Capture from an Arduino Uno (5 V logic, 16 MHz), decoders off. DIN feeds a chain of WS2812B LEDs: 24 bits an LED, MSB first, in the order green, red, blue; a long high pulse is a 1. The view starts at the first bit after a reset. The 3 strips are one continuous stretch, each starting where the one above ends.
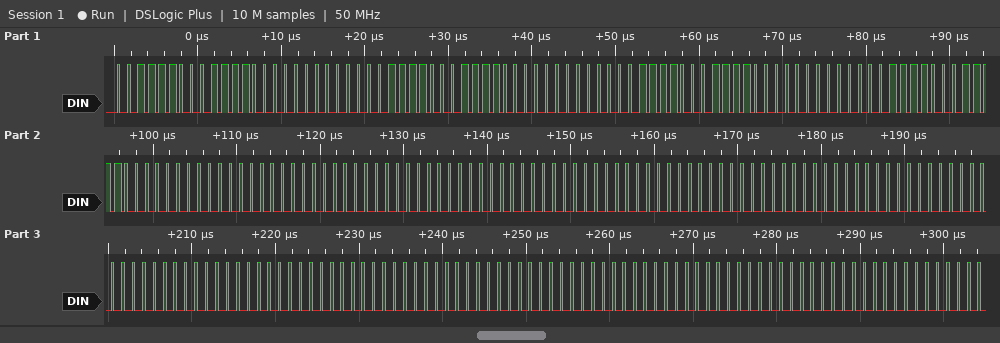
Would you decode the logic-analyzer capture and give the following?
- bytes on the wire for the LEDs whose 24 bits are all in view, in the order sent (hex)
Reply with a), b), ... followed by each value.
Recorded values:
a) 3C 78 00 3C 78 00 3C 78 00 3C 78 00 00 00 00 00 00 00 00 00 00 00 00 00 00 00 00 00 00 00
